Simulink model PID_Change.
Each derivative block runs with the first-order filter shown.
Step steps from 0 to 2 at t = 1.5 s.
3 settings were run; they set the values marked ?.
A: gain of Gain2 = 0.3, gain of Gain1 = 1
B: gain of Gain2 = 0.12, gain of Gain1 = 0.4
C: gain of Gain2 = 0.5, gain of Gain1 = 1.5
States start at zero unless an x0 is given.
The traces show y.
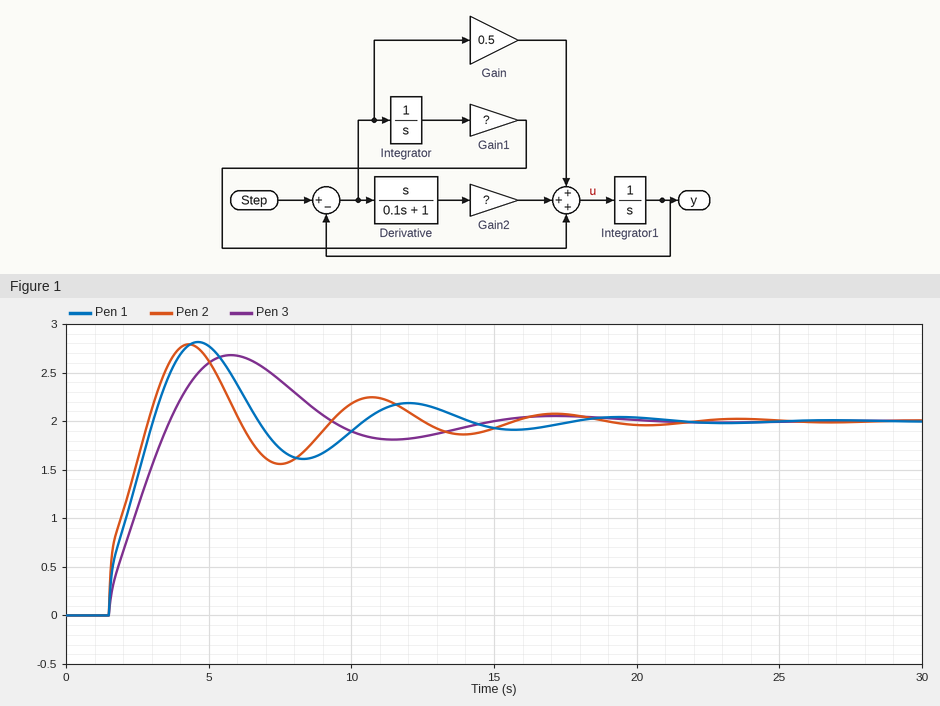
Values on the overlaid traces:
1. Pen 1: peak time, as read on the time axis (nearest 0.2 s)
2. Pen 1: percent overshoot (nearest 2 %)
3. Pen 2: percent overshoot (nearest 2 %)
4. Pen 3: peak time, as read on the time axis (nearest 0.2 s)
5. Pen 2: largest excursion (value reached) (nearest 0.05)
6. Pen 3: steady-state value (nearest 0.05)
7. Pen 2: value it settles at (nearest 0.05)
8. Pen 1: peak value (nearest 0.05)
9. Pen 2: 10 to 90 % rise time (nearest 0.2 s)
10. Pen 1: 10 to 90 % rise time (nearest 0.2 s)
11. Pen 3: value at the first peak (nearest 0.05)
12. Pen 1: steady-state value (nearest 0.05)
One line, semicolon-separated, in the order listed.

4.6 s; 40 %; 40 %; 5.8 s; 2.80; 2.00; 2.00; 2.80; 1.2 s; 1.4 s; 2.70; 2.00
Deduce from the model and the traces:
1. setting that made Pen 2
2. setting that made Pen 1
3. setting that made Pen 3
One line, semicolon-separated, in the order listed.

C; A; B
